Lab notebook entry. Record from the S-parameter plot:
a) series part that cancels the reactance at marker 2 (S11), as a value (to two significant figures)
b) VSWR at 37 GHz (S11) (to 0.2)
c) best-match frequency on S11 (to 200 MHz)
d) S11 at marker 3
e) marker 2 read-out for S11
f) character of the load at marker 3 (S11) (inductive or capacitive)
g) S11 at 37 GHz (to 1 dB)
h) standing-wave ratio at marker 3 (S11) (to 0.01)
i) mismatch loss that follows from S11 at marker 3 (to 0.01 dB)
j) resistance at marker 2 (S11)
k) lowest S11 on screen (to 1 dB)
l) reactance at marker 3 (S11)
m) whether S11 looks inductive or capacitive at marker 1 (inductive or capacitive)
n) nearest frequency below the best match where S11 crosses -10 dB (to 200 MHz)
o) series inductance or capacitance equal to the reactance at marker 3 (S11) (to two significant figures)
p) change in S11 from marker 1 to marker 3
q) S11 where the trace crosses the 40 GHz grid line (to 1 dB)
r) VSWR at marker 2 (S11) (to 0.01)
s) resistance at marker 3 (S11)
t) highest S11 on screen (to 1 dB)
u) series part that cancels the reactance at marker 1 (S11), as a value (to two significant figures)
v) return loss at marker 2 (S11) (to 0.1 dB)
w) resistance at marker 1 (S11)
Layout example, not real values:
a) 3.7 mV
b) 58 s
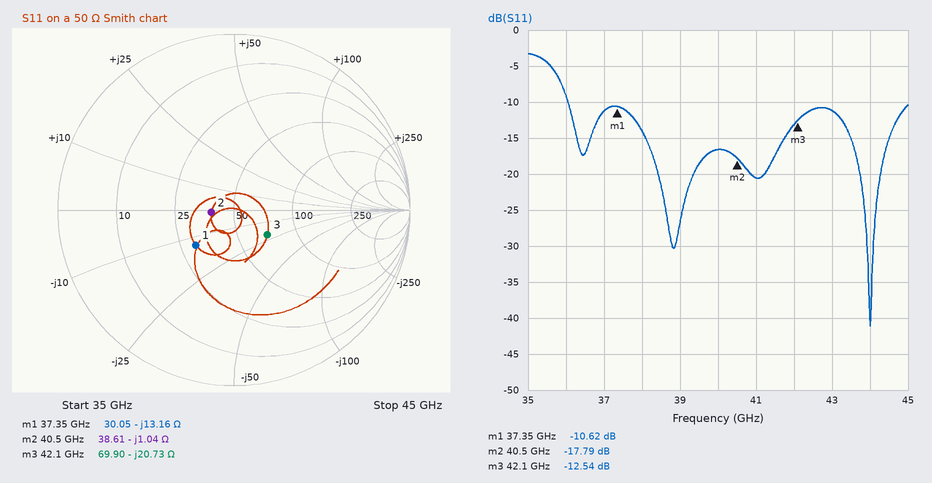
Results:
a) 4.1 pH
b) 1.8
c) 44.0 GHz
d) -12.54 dB
e) -17.79 dB
f) capacitive
g) -11 dB
h) 1.62
i) 0.25 dB
j) 38.61 Ω
k) -41 dB
l) -20.73 Ω
m) capacitive
n) 36.0 GHz
o) 180 fF
p) -1.92 dB
q) -17 dB
r) 1.30
s) 69.90 Ω
t) -3 dB
u) 56 pH
v) 17.8 dB
w) 30.05 Ω
